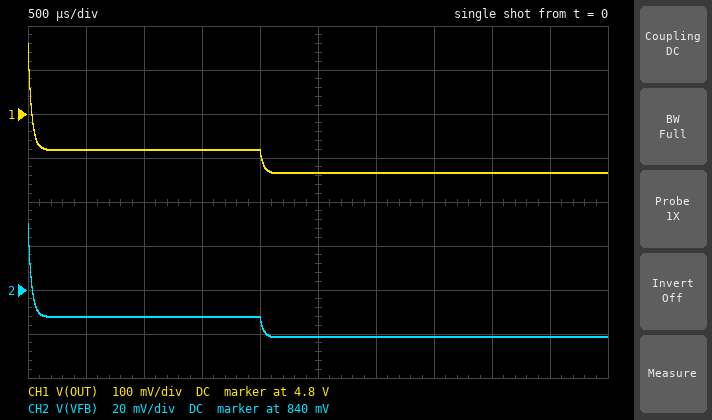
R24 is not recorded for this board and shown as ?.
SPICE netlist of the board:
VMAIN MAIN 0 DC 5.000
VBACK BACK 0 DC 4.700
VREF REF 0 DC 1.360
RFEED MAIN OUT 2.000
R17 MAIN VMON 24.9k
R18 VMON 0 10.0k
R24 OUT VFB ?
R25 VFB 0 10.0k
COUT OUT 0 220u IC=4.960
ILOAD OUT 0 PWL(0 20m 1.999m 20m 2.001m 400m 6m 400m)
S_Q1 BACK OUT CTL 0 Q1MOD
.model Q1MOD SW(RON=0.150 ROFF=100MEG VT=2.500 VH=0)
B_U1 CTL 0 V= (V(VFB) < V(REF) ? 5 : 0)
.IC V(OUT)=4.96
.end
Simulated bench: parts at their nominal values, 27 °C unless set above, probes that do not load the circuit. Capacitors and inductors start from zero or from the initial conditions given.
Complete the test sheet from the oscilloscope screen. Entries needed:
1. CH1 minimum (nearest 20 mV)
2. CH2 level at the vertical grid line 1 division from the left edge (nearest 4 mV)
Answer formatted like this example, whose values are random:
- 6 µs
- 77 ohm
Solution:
- 4.66 V
- 828 mV
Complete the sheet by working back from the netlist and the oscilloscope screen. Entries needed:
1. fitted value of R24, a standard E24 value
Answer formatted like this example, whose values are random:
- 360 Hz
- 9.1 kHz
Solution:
- 47 kΩ
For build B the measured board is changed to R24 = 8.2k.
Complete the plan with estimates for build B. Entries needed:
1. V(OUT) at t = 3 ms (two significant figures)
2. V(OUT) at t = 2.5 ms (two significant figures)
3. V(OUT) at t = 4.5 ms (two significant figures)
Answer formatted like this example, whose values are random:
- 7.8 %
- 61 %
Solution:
- 4.3 V
- 4.4 V
- 4.2 V
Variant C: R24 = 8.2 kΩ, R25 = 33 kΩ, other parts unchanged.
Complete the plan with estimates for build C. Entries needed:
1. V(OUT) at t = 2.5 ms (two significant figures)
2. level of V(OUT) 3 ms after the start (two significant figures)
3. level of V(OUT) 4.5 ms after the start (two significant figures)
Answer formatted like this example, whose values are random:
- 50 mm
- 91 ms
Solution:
- 4.4 V
- 4.3 V
- 4.2 V
